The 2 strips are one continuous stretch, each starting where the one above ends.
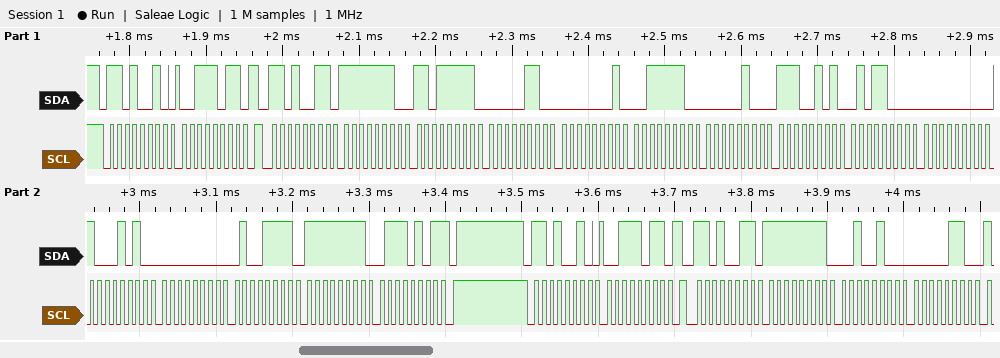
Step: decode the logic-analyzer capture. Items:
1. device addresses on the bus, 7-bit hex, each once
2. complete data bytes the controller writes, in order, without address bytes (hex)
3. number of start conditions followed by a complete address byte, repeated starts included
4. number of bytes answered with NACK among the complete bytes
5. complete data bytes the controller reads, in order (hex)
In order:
0x69
3B 3B
4
1
FE DF 06 01 3E 04 E5 58 00 8A 00 4F FF 75 FF 24 06
